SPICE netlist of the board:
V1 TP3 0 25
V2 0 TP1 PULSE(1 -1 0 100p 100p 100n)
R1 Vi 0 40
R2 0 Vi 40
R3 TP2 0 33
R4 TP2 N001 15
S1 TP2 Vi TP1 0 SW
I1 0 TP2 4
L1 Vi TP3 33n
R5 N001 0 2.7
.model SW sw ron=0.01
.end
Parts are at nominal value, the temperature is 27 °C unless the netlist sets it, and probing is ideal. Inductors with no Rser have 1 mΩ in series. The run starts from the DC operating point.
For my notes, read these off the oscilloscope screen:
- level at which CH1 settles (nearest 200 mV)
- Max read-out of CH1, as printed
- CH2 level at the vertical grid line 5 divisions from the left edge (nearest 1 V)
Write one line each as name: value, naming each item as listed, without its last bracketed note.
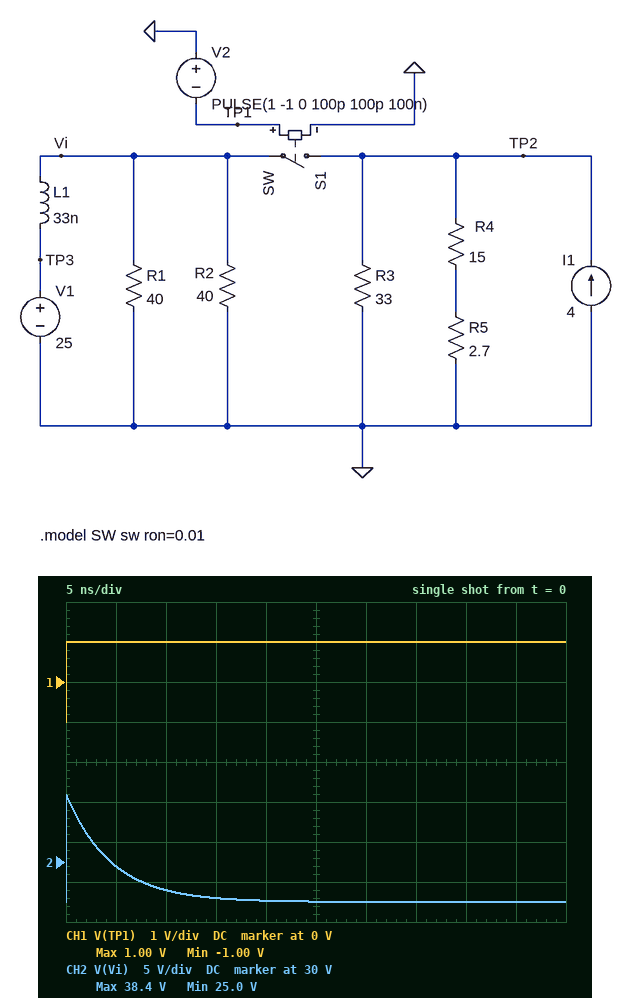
level at which CH1 settles: 1.0 V
Max read-out of CH1, as printed: 1.00 V
CH2 level at the vertical grid line 5 divisions from the left edge: 25 V
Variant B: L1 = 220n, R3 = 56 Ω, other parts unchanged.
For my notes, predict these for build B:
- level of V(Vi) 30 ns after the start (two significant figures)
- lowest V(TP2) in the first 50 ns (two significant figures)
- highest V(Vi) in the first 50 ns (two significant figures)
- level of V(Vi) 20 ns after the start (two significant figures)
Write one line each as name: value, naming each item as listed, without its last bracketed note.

level of V(Vi) 30 ns after the start: 31 V
lowest V(TP2) in the first 50 ns: 28 V
highest V(Vi) in the first 50 ns: 42 V
level of V(Vi) 20 ns after the start: 33 V
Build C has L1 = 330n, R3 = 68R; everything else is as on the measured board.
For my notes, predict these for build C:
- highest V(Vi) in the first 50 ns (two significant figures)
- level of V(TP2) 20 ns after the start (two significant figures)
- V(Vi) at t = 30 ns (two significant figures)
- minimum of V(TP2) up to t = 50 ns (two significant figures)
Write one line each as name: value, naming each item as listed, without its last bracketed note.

highest V(Vi) in the first 50 ns: 43 V
level of V(TP2) 20 ns after the start: 36 V
V(Vi) at t = 30 ns: 34 V
minimum of V(TP2) up to t = 50 ns: 30 V
